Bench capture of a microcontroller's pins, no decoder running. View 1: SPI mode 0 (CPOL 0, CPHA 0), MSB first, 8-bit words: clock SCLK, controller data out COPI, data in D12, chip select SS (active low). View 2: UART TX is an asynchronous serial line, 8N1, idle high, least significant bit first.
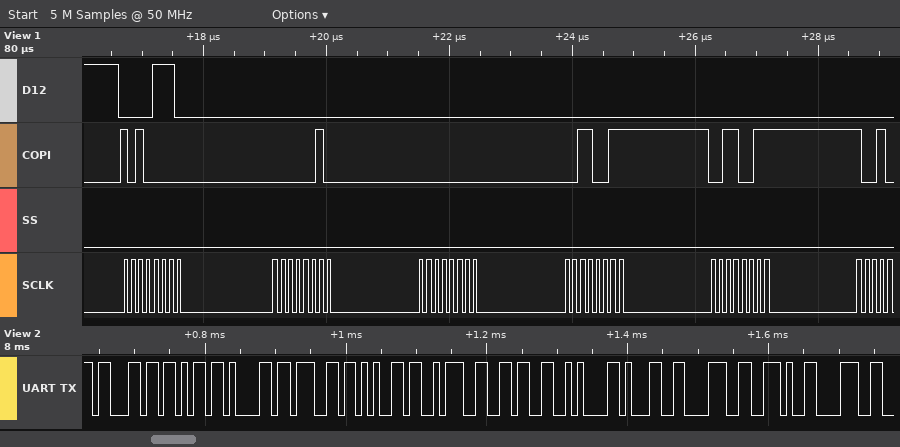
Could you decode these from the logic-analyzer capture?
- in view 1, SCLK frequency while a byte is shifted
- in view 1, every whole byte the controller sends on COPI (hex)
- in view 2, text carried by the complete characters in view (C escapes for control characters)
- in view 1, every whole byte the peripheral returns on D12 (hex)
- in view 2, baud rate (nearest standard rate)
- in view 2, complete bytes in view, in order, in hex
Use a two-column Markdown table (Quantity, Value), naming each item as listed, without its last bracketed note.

| Quantity | Value |
|---|---|
| in view 1, SCLK frequency while a byte is shifted | 8 MHz |
| in view 1, every whole byte the controller sends on COPI | 0xA0 0x02 0x00 0x33 0x33 |
| in view 2, text carried by the complete characters in view | "ckage:6\n18.8" |
| in view 1, every whole byte the peripheral returns on D12 | 0x0E 0x00 0x00 0x00 0x00 |
| in view 2, baud rate | 115200 baud |
| in view 2, complete bytes in view, in order, in hex | 63 6B 61 67 65 3A 36 0A 31 38 2E 38 |
